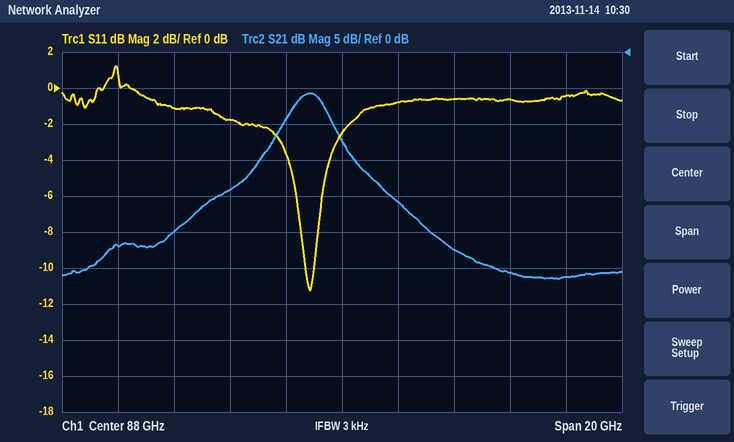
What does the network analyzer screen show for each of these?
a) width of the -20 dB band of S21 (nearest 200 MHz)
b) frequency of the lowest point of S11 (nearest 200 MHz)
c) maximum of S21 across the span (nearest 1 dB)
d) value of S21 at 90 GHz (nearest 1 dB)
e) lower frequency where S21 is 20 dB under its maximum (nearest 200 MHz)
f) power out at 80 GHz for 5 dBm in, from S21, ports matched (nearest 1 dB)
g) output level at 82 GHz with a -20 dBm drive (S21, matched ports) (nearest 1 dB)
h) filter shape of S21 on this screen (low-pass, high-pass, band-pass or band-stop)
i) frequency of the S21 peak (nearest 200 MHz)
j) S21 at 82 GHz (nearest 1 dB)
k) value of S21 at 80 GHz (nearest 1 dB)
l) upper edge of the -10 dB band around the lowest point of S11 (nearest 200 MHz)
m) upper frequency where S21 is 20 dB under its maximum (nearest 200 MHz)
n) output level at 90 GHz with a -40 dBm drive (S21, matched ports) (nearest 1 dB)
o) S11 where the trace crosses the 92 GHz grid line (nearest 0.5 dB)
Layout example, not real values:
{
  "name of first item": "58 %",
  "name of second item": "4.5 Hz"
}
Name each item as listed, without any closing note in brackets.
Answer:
{
  "width of the -20 dB band of S21": "9.6 GHz",
  "frequency of the lowest point of S11": "86.8 GHz",
  "maximum of S21 across the span": "-6 dB",
  "value of S21 at 90 GHz": "-21 dB",
  "lower frequency where S21 is 20 dB under its maximum": "81.8 GHz",
  "power out at 80 GHz for 5 dBm in, from S21, ports matched": "-22 dBm",
  "output level at 82 GHz with a -20 dBm drive (S21, matched ports)": "-45 dBm",
  "filter shape of S21 on this screen": "band-pass",
  "frequency of the S21 peak": "86.8 GHz",
  "S21 at 82 GHz": "-25 dB",
  "value of S21 at 80 GHz": "-27 dB",
  "upper edge of the -10 dB band around the lowest point of S11": "87.0 GHz",
  "upper frequency where S21 is 20 dB under its maximum": "91.4 GHz",
  "output level at 90 GHz with a -40 dBm drive (S21, matched ports)": "-61 dBm",
  "S11 where the trace crosses the 92 GHz grid line": "-0.5 dB"
}
